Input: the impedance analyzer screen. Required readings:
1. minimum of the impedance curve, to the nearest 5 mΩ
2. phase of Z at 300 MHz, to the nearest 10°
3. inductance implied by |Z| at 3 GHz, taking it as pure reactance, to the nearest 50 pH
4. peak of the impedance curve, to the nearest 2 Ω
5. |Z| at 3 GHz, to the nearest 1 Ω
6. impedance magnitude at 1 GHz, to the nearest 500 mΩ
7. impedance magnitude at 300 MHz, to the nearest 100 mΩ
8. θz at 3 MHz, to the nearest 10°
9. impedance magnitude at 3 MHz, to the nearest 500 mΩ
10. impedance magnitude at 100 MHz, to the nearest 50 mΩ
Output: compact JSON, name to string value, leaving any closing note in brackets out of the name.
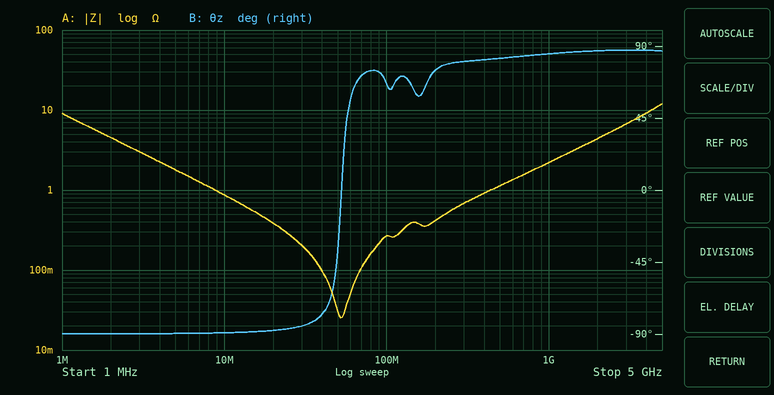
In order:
{"minimum of the impedance curve, to the nearest 5 mΩ": "25 mΩ", "phase of Z at 300 MHz, to the nearest 10°": "80°", "inductance implied by |Z| at 3 GHz, taking it as pure reactance, to the nearest 50 pH": "350 pH", "peak of the impedance curve, to the nearest 2 Ω": "12 Ω", "|Z| at 3 GHz, to the nearest 1 Ω": "7 Ω", "impedance magnitude at 1 GHz, to the nearest 500 mΩ": "2.0 Ω", "impedance magnitude at 300 MHz, to the nearest 100 mΩ": "700 mΩ", "θz at 3 MHz, to the nearest 10°": "-90°", "impedance magnitude at 3 MHz, to the nearest 500 mΩ": "3.0 Ω", "impedance magnitude at 100 MHz, to the nearest 50 mΩ": "250 mΩ"}
